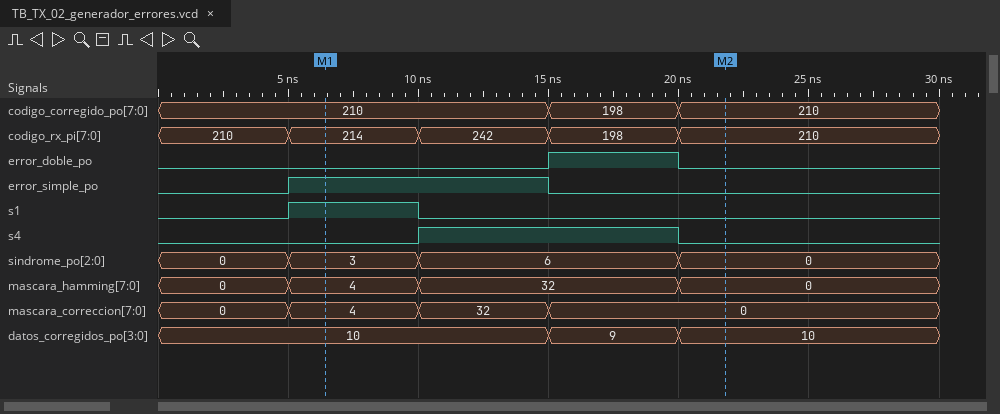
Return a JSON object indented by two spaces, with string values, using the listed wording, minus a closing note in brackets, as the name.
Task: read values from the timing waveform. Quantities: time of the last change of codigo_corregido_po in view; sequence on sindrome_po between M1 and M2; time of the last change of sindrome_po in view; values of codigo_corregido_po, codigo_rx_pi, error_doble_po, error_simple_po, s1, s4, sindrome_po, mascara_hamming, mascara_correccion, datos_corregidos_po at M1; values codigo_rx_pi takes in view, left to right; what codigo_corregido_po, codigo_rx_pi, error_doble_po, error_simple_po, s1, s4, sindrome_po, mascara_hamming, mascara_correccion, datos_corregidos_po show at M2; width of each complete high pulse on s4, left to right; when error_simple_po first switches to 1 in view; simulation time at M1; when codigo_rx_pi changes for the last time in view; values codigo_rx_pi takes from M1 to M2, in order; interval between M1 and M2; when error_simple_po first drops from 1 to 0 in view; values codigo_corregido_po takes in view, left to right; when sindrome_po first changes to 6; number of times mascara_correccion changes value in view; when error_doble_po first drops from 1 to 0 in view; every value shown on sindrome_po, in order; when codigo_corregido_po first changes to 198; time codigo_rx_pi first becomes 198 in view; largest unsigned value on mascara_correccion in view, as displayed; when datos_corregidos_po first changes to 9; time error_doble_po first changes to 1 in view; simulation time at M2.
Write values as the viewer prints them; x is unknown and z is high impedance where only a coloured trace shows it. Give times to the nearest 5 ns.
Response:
{
  "time of the last change of codigo_corregido_po in view": "20 ns",
  "sequence on sindrome_po between M1 and M2": "3, 6, 0",
  "time of the last change of sindrome_po in view": "20 ns",
  "values of codigo_corregido_po, codigo_rx_pi, error_doble_po, error_simple_po, s1, s4, sindrome_po, mascara_hamming, mascara_correccion, datos_corregidos_po at M1": "codigo_corregido_po=210, codigo_rx_pi=214, error_doble_po=0, error_simple_po=1, s1=1, s4=0, sindrome_po=3, mascara_hamming=4, mascara_correccion=4, datos_corregidos_po=10",
  "values codigo_rx_pi takes in view, left to right": "210, 214, 242, 198, 210",
  "what codigo_corregido_po, codigo_rx_pi, error_doble_po, error_simple_po, s1, s4, sindrome_po, mascara_hamming, mascara_correccion, datos_corregidos_po show at M2": "codigo_corregido_po=210, codigo_rx_pi=210, error_doble_po=0, error_simple_po=0, s1=0, s4=0, sindrome_po=0, mascara_hamming=0, mascara_correccion=0, datos_corregidos_po=10",
  "width of each complete high pulse on s4, left to right": "10 ns",
  "when error_simple_po first switches to 1 in view": "5 ns",
  "simulation time at M1": "5 ns",
  "when codigo_rx_pi changes for the last time in view": "20 ns",
  "values codigo_rx_pi takes from M1 to M2, in order": "214, 242, 198, 210",
  "interval between M1 and M2": "15 ns",
  "when error_simple_po first drops from 1 to 0 in view": "15 ns",
  "values codigo_corregido_po takes in view, left to right": "210, 198, 210",
  "when sindrome_po first changes to 6": "10 ns",
  "number of times mascara_correccion changes value in view": "3",
  "when error_doble_po first drops from 1 to 0 in view": "20 ns",
  "every value shown on sindrome_po, in order": "0, 3, 6, 0",
  "when codigo_corregido_po first changes to 198": "15 ns",
  "time codigo_rx_pi first becomes 198 in view": "15 ns",
  "largest unsigned value on mascara_correccion in view, as displayed": "32",
  "when datos_corregidos_po first changes to 9": "15 ns",
  "time error_doble_po first changes to 1 in view": "15 ns",
  "simulation time at M2": "20 ns"
}
